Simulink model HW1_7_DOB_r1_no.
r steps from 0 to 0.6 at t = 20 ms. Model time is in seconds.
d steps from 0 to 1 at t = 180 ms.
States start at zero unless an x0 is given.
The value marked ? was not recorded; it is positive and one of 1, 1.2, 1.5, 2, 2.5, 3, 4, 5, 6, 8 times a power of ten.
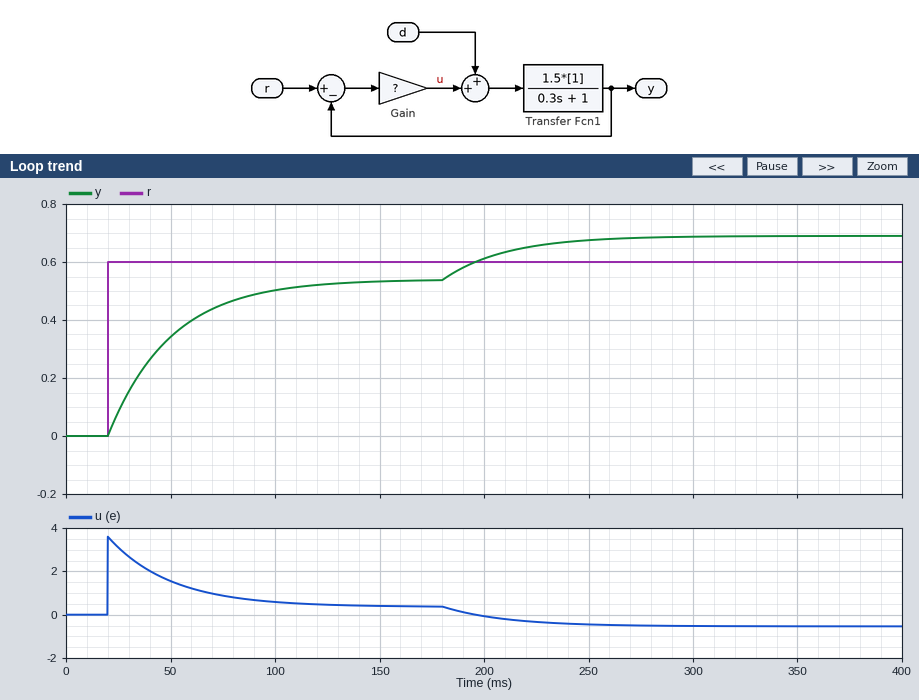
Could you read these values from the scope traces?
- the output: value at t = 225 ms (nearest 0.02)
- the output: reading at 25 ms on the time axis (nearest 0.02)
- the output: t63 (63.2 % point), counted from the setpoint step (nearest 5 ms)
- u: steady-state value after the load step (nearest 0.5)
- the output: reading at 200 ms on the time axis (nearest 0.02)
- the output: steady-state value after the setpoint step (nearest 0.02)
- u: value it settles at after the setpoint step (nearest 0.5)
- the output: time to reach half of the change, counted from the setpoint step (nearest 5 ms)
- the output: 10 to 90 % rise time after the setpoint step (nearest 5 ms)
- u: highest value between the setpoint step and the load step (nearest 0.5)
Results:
0.66
0.08
30 ms
-0.5
0.62
0.54
0.5
20 ms
65 ms
3.5
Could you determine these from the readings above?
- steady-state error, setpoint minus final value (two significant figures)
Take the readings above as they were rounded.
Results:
0.060
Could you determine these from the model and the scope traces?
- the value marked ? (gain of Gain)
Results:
6
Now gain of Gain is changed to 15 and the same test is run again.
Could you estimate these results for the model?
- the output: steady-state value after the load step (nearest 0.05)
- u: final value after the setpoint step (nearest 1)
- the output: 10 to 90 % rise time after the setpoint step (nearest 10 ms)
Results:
0.65
0
30 ms
